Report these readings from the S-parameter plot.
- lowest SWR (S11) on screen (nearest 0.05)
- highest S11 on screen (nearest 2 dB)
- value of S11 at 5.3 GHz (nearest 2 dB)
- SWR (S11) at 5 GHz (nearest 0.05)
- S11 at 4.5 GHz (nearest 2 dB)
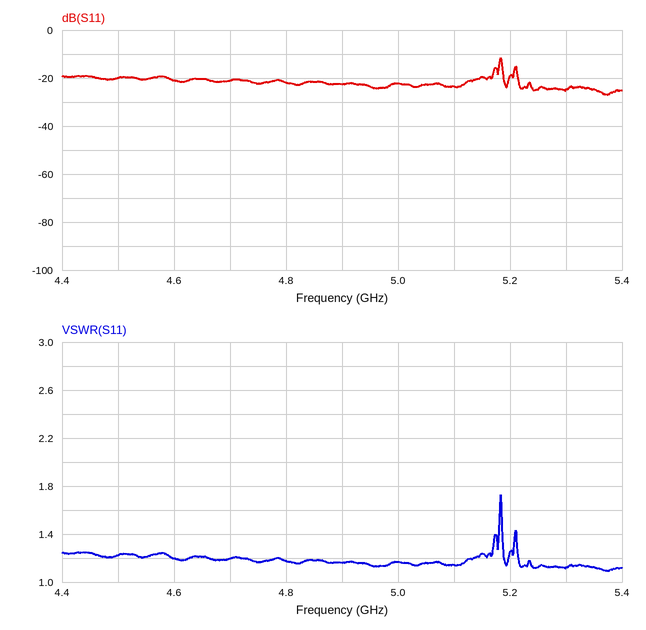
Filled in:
1.10
-12 dB
-24 dB
1.15
-20 dB
